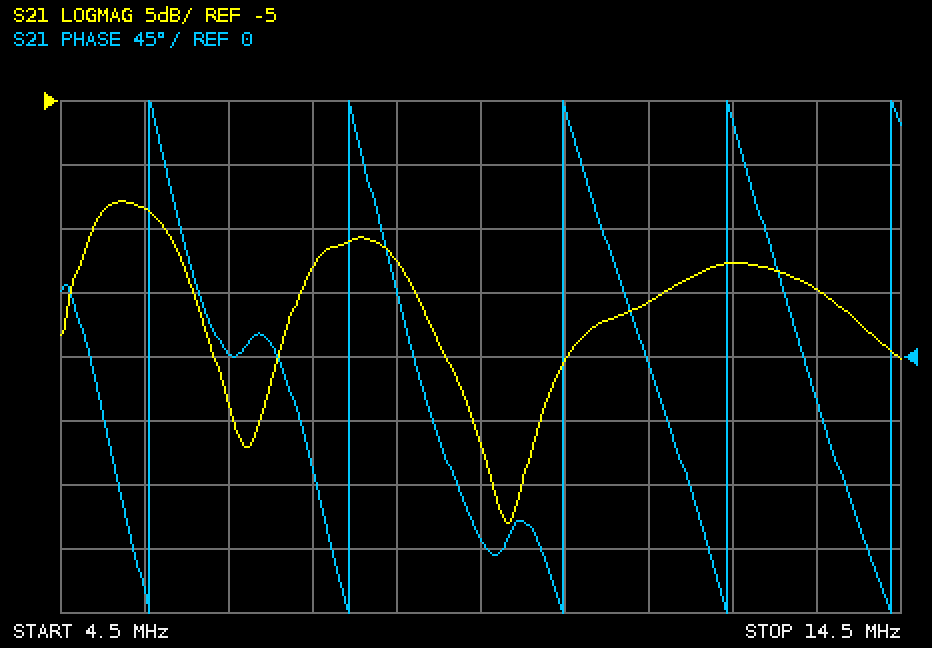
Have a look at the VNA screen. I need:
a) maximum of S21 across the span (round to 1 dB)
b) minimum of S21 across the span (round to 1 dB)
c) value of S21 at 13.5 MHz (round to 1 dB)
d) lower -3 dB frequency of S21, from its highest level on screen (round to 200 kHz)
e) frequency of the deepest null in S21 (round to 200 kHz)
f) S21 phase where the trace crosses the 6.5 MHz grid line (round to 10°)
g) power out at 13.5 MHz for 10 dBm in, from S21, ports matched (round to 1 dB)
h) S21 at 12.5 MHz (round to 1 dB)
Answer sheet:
-13 dB
-38 dB
-20 dB
4.8 MHz
9.8 MHz
0°
-10 dBm
-18 dB
